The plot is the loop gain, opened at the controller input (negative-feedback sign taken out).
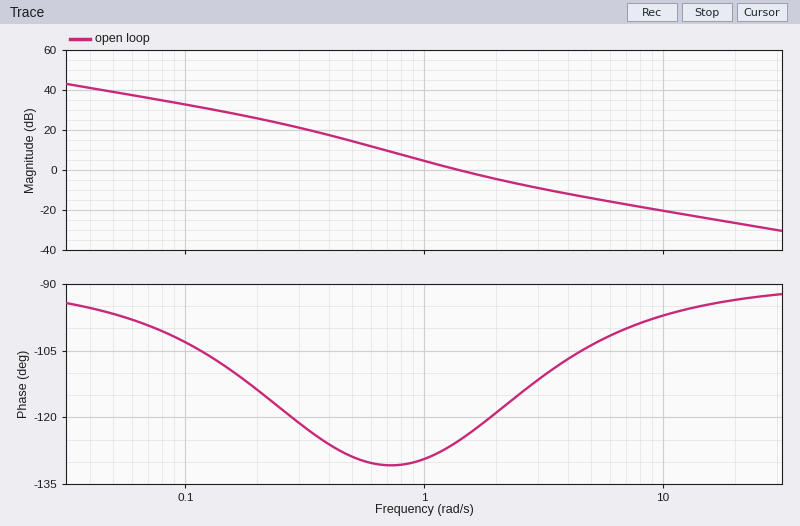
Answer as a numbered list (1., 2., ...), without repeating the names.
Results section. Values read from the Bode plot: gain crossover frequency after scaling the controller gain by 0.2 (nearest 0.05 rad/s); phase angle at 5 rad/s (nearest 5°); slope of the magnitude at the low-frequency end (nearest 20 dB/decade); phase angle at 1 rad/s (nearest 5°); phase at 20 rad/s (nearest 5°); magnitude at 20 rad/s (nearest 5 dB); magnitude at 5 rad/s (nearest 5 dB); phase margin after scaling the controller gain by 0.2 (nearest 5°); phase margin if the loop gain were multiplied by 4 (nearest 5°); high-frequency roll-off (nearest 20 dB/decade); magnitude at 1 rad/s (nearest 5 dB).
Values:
1. 0.50 rad/s
2. -105°
3. -20 dB/decade
4. -130°
5. -95°
6. -25 dB
7. -15 dB
8. 50°
9. 75°
10. -20 dB/decade
11. 5 dB
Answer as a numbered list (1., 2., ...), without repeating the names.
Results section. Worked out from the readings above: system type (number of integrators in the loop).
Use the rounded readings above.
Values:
1. 1
